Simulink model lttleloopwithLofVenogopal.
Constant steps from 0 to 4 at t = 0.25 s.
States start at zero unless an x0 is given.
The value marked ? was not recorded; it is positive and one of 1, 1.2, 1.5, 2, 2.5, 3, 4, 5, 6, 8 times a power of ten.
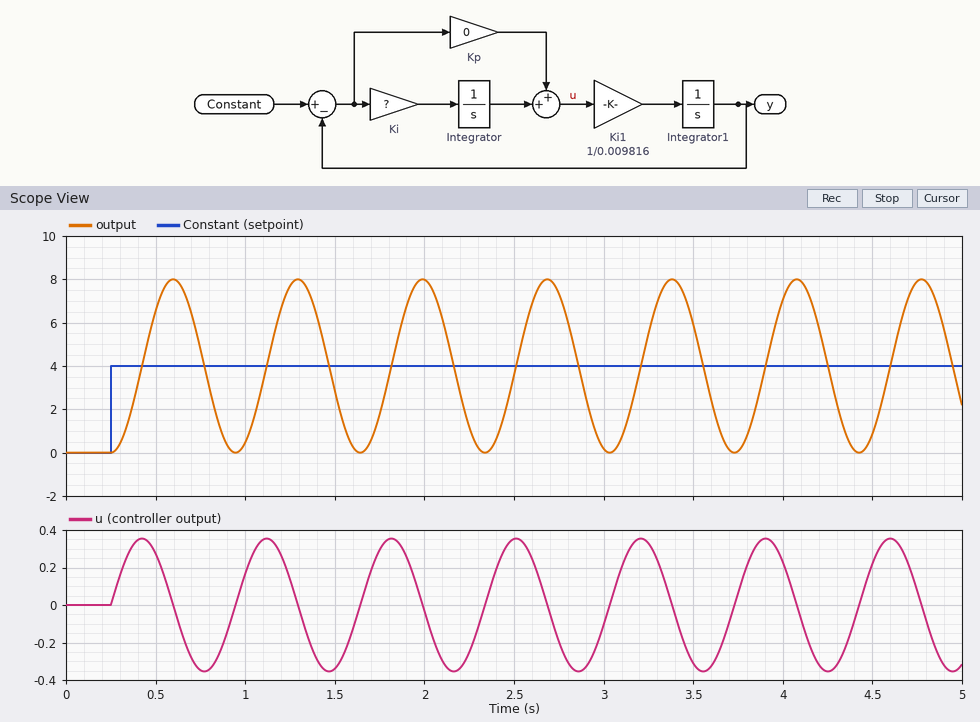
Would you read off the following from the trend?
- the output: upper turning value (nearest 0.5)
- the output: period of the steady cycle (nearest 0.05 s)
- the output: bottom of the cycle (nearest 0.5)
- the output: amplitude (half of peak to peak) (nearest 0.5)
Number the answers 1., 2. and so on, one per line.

1. 8.0
2. 0.70 s
3. 0.0
4. 4.0
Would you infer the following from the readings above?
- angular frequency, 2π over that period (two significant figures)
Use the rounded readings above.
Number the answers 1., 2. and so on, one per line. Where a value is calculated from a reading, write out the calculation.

1. 2π / 0.7 = 9.0 rad/s
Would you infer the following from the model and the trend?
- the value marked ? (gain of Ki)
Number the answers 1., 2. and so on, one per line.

1. 0.8
